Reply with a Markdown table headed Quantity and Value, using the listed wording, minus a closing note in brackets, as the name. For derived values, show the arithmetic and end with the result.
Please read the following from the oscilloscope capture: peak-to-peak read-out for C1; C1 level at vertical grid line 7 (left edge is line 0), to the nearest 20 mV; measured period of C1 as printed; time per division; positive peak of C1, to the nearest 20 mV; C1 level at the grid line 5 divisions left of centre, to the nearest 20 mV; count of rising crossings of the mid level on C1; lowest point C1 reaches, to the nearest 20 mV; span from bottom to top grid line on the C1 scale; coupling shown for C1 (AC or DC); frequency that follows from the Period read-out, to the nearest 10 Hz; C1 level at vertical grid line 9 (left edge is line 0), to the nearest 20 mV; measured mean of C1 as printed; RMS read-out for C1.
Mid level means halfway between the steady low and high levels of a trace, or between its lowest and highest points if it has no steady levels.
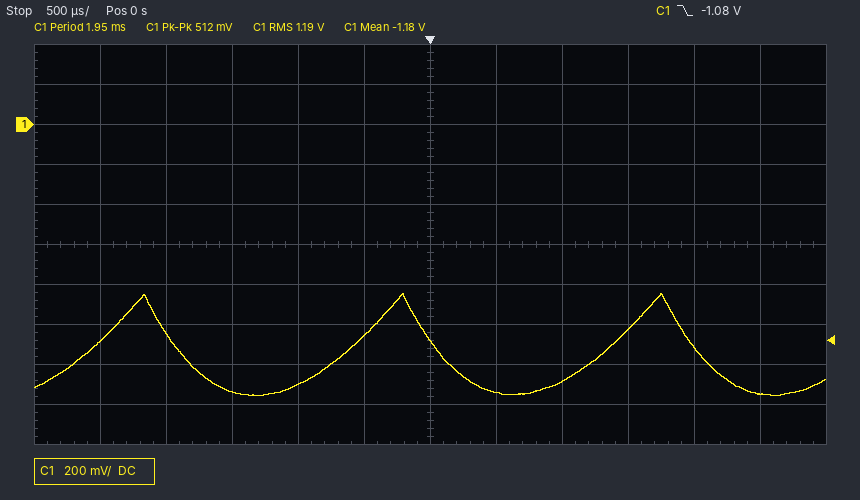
| Quantity | Value |
|---|---|
| peak-to-peak read-out for C1 | 512 mV |
| C1 level at vertical grid line 7 (left edge is line 0), to the nearest 20 mV | -1.34 V |
| measured period of C1 as printed | 1.95 ms |
| time per division | 500 µs |
| positive peak of C1, to the nearest 20 mV | -840 mV |
| C1 level at the grid line 5 divisions left of centre, to the nearest 20 mV | -1.08 V |
| count of rising crossings of the mid level on C1 | 3 |
| lowest point C1 reaches, to the nearest 20 mV | -1.36 V |
| span from bottom to top grid line on the C1 scale | 2 V |
| coupling shown for C1 | DC |
| frequency that follows from the Period read-out, to the nearest 10 Hz | 1 / 1.95 ms ≈ 513 Hz, so 510 Hz to the nearest 10 Hz |
| C1 level at vertical grid line 9 (left edge is line 0), to the nearest 20 mV | -1.02 V |
| measured mean of C1 as printed | -1.18 V |
| RMS read-out for C1 | 1.19 V |
